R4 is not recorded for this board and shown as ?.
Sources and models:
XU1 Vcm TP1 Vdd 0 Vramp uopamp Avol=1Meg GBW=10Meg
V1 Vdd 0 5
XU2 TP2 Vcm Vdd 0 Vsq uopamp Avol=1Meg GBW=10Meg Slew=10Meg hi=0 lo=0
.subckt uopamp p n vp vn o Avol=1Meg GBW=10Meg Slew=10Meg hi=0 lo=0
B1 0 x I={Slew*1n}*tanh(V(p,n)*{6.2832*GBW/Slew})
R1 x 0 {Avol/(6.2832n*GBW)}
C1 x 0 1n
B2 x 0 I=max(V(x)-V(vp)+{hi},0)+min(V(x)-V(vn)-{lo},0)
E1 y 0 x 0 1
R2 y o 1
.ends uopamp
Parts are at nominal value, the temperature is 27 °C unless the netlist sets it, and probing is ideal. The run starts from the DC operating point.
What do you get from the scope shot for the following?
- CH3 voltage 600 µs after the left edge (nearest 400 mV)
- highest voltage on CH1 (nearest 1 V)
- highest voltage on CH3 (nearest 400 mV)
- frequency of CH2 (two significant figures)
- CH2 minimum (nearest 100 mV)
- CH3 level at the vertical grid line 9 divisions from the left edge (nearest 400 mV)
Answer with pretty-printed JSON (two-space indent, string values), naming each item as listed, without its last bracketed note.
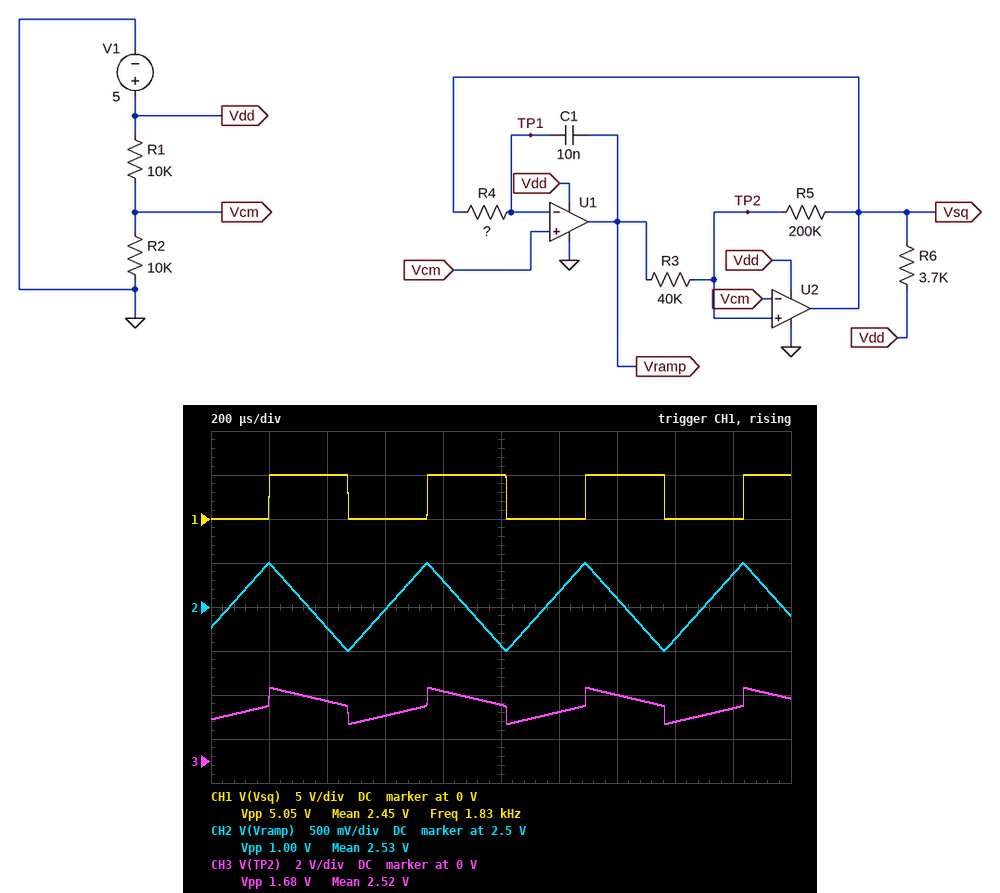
{
  "CH3 voltage 600 µs after the left edge": "2.0 V",
  "highest voltage on CH1": "5 V",
  "highest voltage on CH3": "3.2 V",
  "frequency of CH2": "1.8 kHz",
  "CH2 minimum": "2.0 V",
  "CH3 level at the vertical grid line 9 divisions from the left edge": "2.4 V"
}
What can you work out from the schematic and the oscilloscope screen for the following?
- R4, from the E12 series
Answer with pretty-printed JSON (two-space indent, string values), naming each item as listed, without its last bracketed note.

{
  "R4, from the E12 series": "68 kΩ"
}
